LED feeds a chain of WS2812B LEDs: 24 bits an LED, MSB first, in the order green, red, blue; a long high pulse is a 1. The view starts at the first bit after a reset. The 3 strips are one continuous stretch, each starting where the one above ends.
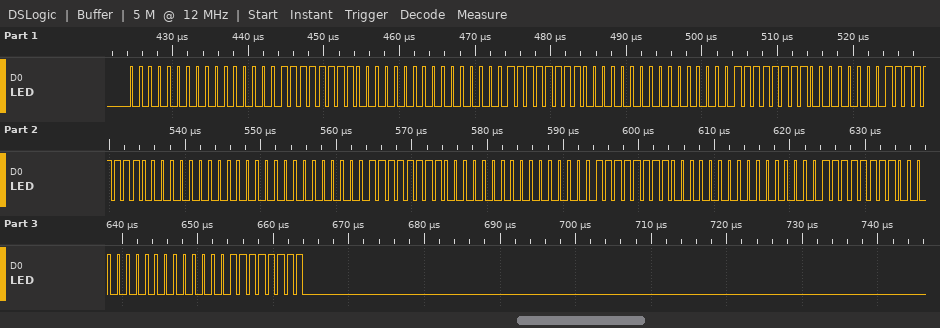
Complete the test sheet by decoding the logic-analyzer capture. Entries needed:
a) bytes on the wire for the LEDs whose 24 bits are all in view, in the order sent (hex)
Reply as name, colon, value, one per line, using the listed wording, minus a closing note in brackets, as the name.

bytes on the wire for the LEDs whose 24 bits are all in view, in the order sent: 00 00 FF 00 00 FF 00 00 FF 00 FF 00 00 00 FF 00 00 FF 00 00 FF 00 00 FF
